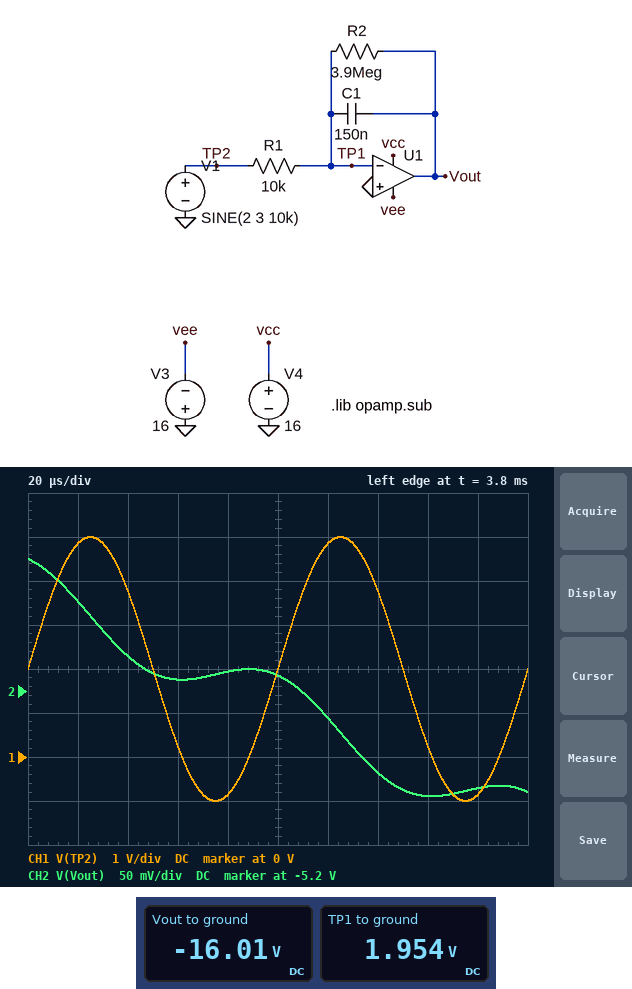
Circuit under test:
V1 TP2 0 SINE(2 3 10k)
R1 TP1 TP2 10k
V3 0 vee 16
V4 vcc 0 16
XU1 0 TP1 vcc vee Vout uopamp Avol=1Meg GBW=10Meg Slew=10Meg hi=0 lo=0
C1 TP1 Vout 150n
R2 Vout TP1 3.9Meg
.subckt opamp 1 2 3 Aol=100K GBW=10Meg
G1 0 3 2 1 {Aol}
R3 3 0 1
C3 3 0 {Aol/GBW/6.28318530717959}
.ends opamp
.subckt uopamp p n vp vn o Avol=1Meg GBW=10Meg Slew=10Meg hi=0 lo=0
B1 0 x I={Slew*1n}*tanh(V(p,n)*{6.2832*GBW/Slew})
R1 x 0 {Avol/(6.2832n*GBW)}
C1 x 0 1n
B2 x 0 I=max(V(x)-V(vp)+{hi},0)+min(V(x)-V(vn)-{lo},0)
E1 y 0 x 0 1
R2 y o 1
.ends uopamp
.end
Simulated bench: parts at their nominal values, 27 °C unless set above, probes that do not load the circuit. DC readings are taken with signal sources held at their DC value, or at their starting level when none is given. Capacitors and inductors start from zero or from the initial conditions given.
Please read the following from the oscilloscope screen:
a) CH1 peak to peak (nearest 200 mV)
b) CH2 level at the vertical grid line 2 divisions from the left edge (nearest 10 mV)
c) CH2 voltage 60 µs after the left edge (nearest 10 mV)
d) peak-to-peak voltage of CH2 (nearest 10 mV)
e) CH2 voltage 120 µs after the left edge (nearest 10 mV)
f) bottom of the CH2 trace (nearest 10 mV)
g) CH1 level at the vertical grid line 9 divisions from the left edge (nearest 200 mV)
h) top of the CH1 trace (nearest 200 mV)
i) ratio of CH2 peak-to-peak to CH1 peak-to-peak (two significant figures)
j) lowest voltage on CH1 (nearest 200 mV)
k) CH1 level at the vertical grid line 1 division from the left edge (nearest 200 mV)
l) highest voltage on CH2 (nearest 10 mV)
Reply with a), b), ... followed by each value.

a) 6.0 V
b) -5.16 V
c) -5.19 V
d) 270 mV
e) -5.23 V
f) -5.32 V
g) -800 mV
h) 5.0 V
i) 0.045
j) -1.0 V
k) 4.8 V
l) -5.05 V
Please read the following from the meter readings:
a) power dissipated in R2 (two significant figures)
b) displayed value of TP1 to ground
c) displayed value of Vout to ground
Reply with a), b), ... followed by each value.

a) 83 µW
b) 1.954 V
c) -16.01 V
